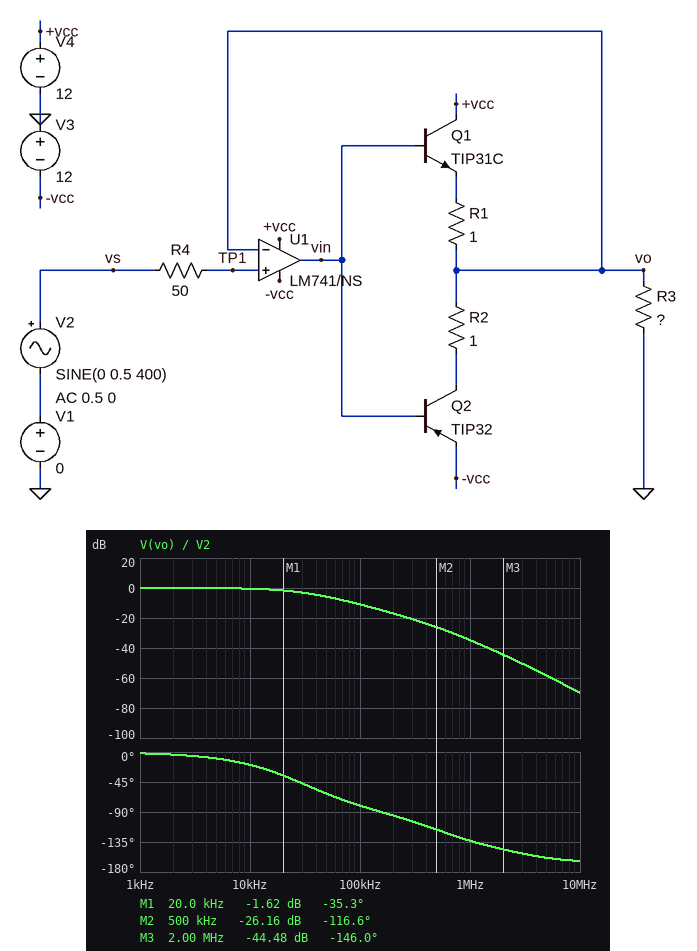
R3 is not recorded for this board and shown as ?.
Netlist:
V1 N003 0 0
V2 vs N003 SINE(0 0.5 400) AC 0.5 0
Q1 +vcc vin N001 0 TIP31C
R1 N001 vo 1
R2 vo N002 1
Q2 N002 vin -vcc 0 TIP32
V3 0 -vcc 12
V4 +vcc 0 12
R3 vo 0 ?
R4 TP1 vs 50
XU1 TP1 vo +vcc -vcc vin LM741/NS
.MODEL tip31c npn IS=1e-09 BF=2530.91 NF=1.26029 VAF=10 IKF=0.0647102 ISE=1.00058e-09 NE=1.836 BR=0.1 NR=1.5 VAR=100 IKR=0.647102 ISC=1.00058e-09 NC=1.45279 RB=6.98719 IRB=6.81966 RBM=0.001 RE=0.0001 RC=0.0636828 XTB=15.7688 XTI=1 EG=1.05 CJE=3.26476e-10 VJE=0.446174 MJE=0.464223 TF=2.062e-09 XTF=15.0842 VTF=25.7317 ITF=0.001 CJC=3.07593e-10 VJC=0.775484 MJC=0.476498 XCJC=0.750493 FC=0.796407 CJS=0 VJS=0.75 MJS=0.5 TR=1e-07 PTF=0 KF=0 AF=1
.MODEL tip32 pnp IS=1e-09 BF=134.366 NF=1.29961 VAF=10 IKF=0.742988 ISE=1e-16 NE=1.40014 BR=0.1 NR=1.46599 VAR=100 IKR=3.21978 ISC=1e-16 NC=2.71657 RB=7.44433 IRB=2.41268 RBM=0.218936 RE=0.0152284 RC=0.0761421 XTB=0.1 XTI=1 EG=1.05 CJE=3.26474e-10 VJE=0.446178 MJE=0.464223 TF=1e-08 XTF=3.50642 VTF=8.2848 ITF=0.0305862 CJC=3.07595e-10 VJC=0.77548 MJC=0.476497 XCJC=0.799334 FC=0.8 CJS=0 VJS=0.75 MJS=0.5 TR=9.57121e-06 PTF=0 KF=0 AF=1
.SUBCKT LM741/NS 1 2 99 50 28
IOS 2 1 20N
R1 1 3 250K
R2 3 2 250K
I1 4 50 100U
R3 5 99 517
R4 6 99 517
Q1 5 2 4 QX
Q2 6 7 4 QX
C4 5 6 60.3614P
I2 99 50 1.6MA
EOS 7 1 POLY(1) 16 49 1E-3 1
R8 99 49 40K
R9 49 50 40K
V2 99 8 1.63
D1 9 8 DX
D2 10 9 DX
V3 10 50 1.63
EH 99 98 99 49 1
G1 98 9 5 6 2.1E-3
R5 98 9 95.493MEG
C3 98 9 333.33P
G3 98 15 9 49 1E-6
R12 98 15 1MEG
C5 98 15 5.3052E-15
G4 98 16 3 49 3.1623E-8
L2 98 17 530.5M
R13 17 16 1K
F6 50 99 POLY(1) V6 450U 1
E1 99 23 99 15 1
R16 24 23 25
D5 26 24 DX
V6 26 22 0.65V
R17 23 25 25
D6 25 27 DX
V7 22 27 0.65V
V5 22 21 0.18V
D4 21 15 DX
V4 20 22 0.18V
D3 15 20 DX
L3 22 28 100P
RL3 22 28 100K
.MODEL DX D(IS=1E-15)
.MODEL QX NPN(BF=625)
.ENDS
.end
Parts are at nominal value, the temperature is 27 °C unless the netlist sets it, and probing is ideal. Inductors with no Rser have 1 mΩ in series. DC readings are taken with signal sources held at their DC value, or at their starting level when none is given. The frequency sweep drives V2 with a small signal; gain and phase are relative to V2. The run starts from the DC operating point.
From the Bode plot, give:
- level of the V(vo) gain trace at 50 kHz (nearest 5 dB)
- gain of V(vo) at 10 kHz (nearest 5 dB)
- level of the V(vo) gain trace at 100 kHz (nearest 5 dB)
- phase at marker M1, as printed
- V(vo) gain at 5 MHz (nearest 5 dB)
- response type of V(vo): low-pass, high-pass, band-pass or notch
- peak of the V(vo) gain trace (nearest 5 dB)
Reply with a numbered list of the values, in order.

1. -5 dB
2. 0 dB
3. -10 dB
4. -35.3 deg
5. -60 dB
6. low-pass
7. 0 dB
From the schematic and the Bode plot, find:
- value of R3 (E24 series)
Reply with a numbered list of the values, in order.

1. 2.7 Ω
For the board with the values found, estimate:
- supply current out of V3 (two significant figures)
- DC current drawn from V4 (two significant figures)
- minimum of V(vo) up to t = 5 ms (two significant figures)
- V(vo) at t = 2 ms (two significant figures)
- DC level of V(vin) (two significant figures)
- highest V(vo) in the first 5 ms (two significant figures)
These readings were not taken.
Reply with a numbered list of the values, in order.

1. 1.6 mA
2. 2.0 mA
3. -75 mV
4. -75 mV
5. 390 mV
6. 500 mV
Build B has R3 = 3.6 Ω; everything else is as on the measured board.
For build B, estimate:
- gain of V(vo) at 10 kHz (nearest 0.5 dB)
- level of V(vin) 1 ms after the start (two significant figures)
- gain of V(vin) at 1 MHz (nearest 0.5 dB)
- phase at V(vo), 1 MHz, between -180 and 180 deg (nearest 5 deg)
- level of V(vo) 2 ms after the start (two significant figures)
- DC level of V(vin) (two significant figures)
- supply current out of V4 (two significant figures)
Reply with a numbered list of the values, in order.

1. -0.5 dB
2. 960 mV
3. -5.0 dB
4. -125 deg
5. -100 mV
6. 380 mV
7. 1.9 mA
